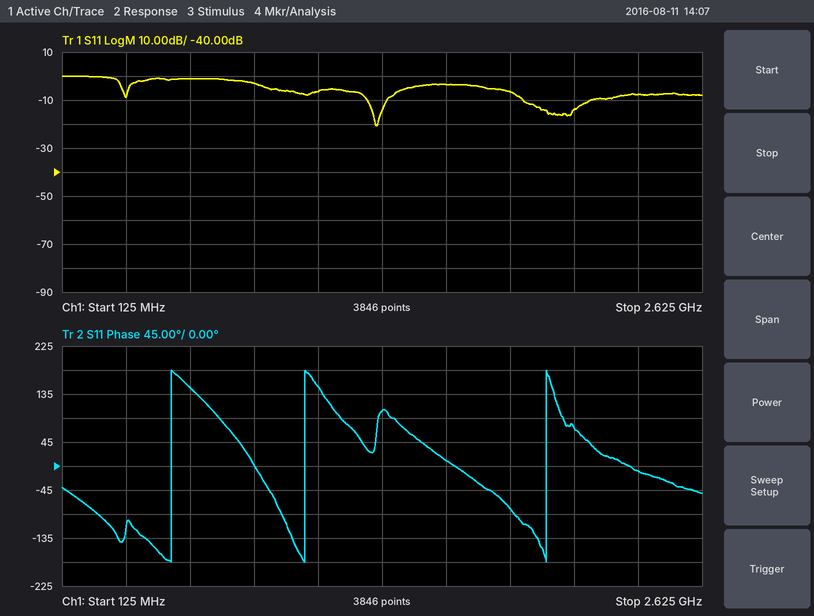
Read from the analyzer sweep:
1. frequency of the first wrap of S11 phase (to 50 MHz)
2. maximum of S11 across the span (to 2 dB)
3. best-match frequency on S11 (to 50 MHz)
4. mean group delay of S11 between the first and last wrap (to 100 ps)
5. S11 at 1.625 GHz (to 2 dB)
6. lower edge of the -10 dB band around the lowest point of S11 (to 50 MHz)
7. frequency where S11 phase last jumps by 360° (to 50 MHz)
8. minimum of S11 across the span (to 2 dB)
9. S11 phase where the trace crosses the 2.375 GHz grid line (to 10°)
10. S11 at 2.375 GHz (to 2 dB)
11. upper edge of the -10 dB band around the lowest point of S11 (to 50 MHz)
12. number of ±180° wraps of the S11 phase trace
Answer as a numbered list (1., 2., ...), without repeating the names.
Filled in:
1. 550 MHz
2. 0 dB
3. 1.35 GHz
4. 1.4 ns
5. -4 dB
6. 1.30 GHz
7. 2.00 GHz
8. -20 dB
9. -10°
10. -8 dB
11. 1.40 GHz
12. 3
